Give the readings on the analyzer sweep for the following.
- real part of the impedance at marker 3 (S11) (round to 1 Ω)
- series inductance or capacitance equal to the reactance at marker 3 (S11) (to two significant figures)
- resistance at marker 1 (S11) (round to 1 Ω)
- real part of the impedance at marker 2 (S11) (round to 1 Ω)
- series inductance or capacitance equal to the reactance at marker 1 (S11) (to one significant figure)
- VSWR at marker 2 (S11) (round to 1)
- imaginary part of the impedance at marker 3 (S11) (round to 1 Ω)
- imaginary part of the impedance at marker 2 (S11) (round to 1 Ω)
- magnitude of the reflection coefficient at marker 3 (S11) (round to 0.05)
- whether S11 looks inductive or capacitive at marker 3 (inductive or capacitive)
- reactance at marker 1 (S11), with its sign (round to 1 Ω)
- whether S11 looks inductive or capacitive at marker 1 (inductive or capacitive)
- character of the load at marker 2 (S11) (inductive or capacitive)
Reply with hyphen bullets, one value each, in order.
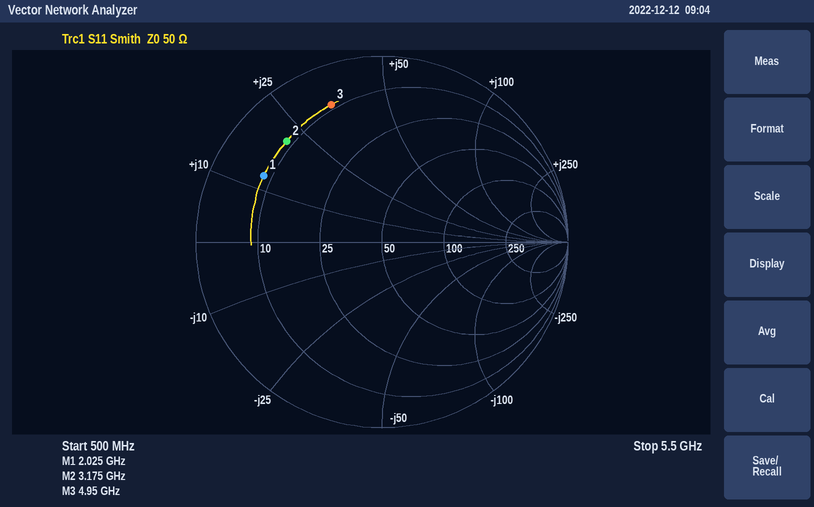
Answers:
- 9 Ω
- 1.1 nH
- 8 Ω
- 9 Ω
- 1.0 nH
- 7
- +34 Ω
- +21 Ω
- 0.80
- inductive
- +13 Ω
- inductive
- inductive
